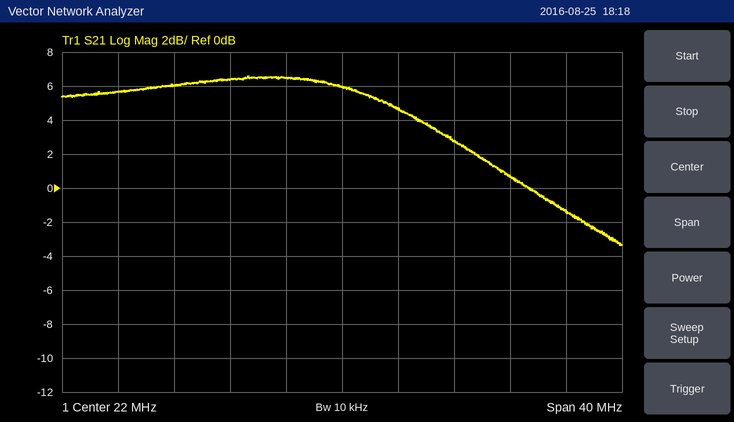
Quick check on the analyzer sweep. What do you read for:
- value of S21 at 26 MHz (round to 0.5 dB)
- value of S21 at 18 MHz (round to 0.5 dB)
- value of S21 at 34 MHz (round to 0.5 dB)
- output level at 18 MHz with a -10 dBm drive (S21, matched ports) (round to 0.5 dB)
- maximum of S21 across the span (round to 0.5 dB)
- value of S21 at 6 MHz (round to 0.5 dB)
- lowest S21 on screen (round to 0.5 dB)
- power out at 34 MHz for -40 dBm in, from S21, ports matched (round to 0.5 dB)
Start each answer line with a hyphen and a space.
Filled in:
- 4.5 dB
- 6.5 dB
- 0.5 dB
- -3.5 dBm
- 6.5 dB
- 5.5 dB
- -3.5 dB
- -39.5 dBm
